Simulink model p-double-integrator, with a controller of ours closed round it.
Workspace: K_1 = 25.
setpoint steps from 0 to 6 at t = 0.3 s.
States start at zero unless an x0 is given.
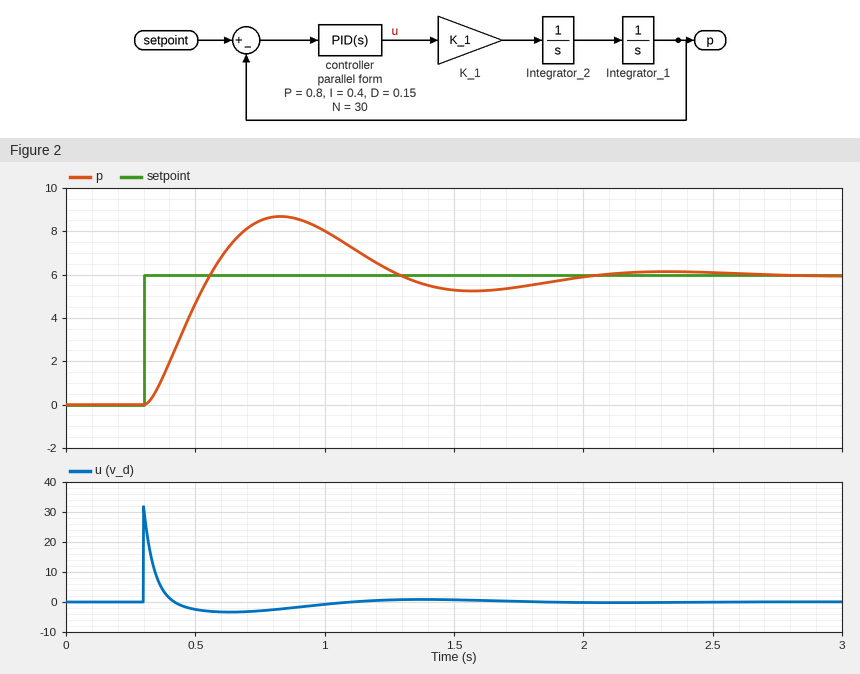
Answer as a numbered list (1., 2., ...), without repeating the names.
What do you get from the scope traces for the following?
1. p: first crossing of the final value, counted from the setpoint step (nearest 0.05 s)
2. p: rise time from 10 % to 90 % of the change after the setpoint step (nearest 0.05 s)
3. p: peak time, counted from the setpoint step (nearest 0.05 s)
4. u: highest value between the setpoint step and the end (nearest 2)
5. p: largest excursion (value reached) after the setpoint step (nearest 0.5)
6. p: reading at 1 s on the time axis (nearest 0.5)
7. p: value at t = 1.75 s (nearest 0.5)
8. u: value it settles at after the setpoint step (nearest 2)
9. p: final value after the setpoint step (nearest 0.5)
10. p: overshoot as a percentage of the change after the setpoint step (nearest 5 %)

1. 0.25 s
2. 0.20 s
3. 0.55 s
4. 32
5. 8.5
6. 8.0
7. 5.5
8. 0
9. 6.0
10. 45 %
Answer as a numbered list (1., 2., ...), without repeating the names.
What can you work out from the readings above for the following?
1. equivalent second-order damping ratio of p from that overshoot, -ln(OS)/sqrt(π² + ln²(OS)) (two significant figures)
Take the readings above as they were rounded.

1. 0.25
